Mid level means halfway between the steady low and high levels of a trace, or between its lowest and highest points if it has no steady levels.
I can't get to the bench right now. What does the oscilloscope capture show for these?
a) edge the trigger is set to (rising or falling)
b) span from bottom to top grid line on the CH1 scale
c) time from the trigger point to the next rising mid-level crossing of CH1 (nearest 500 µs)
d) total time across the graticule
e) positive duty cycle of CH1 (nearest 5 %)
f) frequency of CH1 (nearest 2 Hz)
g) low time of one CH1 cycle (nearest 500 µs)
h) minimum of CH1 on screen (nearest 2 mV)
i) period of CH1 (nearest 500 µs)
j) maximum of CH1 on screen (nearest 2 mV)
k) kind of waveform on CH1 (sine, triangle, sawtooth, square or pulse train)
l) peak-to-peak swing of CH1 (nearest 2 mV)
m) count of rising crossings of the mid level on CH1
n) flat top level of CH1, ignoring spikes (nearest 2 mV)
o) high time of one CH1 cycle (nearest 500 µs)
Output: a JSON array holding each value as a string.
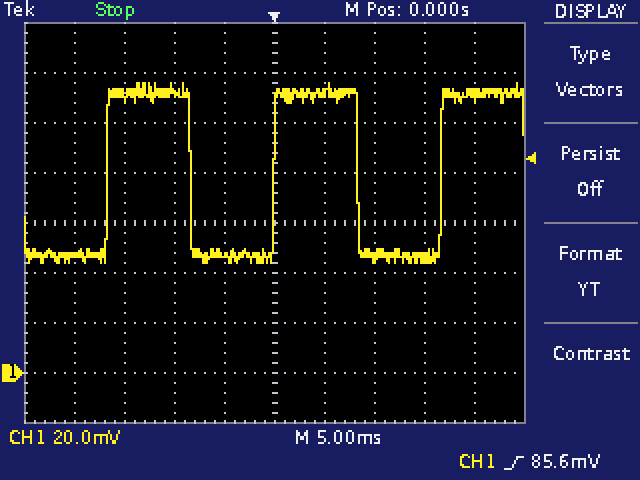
["rising", "160 mV", "16.5 ms", "50 ms", "50 %", "60 Hz", "8.5 ms", "44 mV", "16.5 ms", "116 mV", "square", "72 mV", "3", "112 mV", "8.5 ms"]
